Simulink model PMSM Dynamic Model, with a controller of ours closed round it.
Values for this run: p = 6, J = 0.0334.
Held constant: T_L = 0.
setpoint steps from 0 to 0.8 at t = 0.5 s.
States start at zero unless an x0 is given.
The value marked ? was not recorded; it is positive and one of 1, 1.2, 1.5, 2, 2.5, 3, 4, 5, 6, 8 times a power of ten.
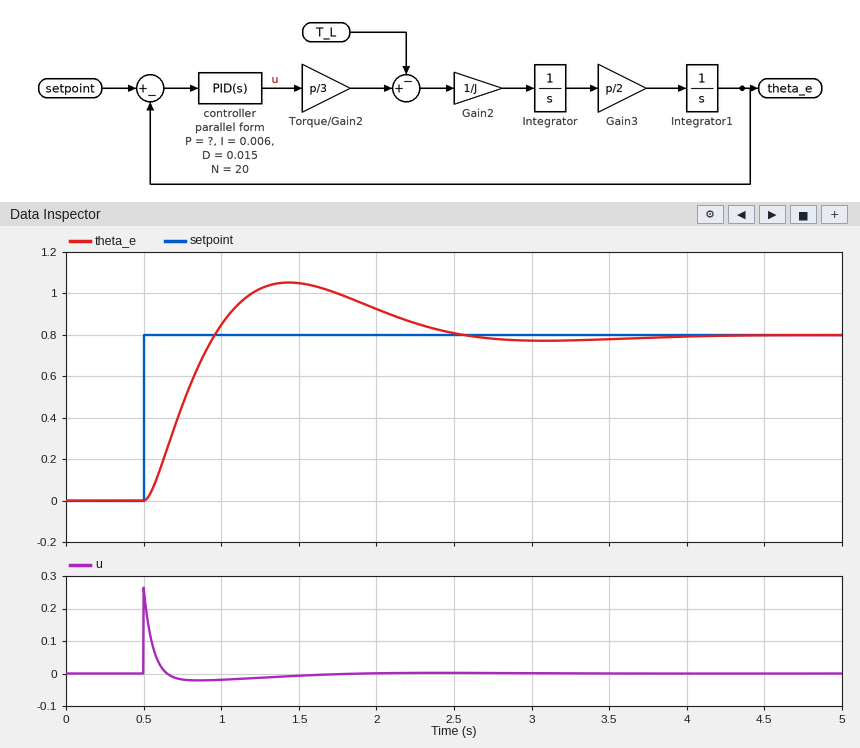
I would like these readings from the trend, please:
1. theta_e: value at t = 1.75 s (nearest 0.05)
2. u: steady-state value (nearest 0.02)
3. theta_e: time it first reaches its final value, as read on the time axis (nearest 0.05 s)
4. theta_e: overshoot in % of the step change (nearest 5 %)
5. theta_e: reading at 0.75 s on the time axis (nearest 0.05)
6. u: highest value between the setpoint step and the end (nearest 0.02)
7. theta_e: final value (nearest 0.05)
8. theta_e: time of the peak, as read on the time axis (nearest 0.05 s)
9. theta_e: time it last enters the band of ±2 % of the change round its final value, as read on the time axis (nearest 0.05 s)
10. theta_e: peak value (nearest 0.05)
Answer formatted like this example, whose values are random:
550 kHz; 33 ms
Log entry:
1.00; 0.00; 0.95 s; 30 %; 0.45; 0.26; 0.80; 1.45 s; 3.65 s; 1.05
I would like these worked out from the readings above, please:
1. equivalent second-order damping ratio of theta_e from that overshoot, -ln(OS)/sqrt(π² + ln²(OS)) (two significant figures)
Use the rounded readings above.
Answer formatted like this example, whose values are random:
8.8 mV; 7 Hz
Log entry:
0.36
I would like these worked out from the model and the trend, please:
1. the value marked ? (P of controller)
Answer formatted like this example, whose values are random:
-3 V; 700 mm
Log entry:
0.03
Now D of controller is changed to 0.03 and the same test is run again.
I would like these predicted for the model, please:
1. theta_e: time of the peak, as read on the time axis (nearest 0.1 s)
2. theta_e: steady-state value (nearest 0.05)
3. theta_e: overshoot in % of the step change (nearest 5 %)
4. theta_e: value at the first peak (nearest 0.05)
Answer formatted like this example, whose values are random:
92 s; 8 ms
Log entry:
1.1 s; 0.80; 15 %; 0.90
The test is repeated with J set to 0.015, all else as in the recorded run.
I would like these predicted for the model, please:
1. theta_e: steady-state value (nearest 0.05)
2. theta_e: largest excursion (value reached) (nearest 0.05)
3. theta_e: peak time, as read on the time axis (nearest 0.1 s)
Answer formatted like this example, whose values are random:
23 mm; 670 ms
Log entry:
0.80; 1.00; 1.0 s
